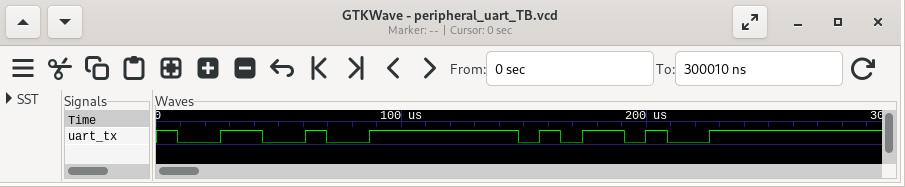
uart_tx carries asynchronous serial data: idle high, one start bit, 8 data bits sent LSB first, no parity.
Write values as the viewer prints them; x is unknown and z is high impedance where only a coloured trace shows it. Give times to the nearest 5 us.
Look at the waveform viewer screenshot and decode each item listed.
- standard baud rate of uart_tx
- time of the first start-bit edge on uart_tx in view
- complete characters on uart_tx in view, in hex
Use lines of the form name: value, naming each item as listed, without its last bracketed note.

standard baud rate of uart_tx: 115200 baud
time of the first start-bit edge on uart_tx in view: 10 us
complete characters on uart_tx in view, in hex: 26, 2D
